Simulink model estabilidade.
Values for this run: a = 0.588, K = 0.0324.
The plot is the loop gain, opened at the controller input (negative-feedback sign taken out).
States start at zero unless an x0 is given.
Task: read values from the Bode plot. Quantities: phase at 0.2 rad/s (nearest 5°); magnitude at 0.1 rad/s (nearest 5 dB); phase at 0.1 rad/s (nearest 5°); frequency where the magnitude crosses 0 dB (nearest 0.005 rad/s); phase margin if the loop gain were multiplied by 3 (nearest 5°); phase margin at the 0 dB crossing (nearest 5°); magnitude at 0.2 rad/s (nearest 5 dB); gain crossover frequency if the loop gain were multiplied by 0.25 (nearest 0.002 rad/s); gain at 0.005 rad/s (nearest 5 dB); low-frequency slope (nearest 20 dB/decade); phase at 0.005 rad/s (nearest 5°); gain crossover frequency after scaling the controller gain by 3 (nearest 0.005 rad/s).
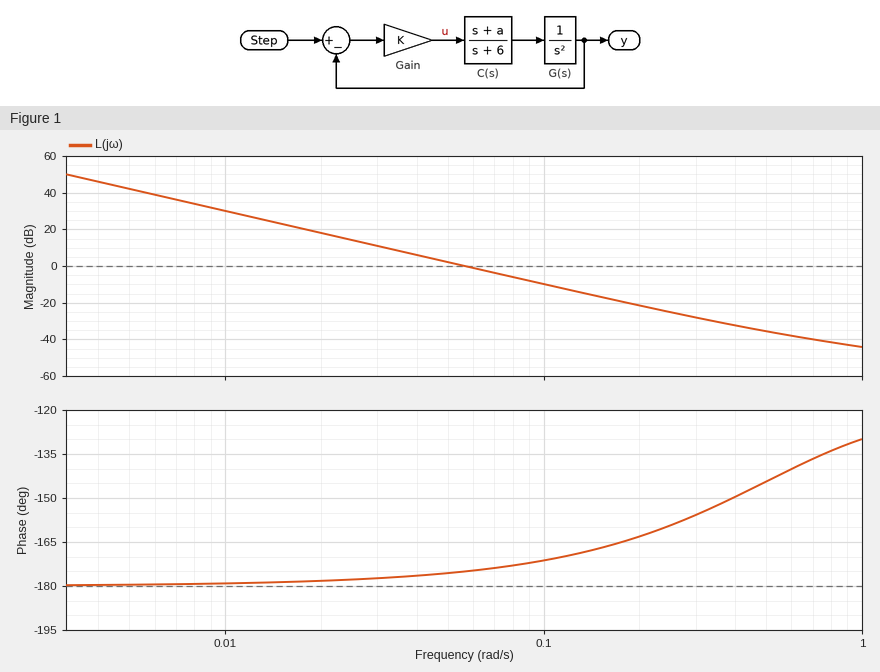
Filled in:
-165°
-10 dB
-170°
0.055 rad/s
10°
5°
-20 dB
0.028 rad/s
40 dB
-40 dB/decade
-180°
0.100 rad/s
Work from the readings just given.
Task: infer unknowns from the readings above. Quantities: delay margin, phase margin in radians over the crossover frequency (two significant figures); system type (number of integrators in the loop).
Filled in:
1.6 s
2
